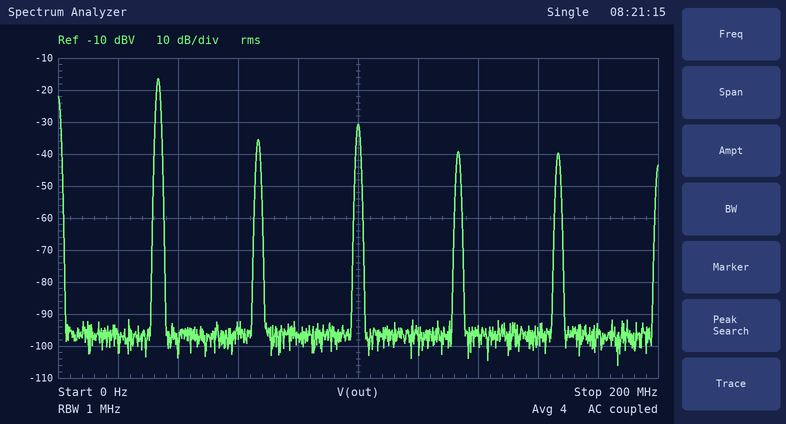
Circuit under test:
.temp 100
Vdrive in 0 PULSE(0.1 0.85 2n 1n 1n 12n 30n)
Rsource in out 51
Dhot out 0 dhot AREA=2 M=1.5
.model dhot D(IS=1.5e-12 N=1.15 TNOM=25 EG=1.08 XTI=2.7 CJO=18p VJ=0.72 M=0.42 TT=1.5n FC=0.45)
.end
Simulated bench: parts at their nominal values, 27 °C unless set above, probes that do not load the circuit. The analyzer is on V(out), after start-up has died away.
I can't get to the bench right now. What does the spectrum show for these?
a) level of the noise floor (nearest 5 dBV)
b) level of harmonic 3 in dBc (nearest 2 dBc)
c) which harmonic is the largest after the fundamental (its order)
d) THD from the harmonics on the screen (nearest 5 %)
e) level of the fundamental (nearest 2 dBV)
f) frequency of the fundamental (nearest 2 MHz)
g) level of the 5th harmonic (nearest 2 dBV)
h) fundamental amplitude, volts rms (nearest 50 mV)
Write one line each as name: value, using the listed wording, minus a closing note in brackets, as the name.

level of the noise floor: -95 dBV
level of harmonic 3 in dBc: -14 dBc
which harmonic is the largest after the fundamental: 3
THD from the harmonics on the screen: 25 %
level of the fundamental: -16 dBV
frequency of the fundamental: 34 MHz
level of the 5th harmonic: -40 dBV
fundamental amplitude, volts rms: 150 mV
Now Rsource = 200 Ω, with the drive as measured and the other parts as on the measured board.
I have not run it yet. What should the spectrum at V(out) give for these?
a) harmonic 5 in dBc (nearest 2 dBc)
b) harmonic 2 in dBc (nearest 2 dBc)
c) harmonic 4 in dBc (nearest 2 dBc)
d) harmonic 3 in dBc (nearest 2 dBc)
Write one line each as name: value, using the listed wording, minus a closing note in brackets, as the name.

harmonic 5 in dBc: -32 dBc
harmonic 2 in dBc: -16 dBc
harmonic 4 in dBc: -26 dBc
harmonic 3 in dBc: -20 dBc
